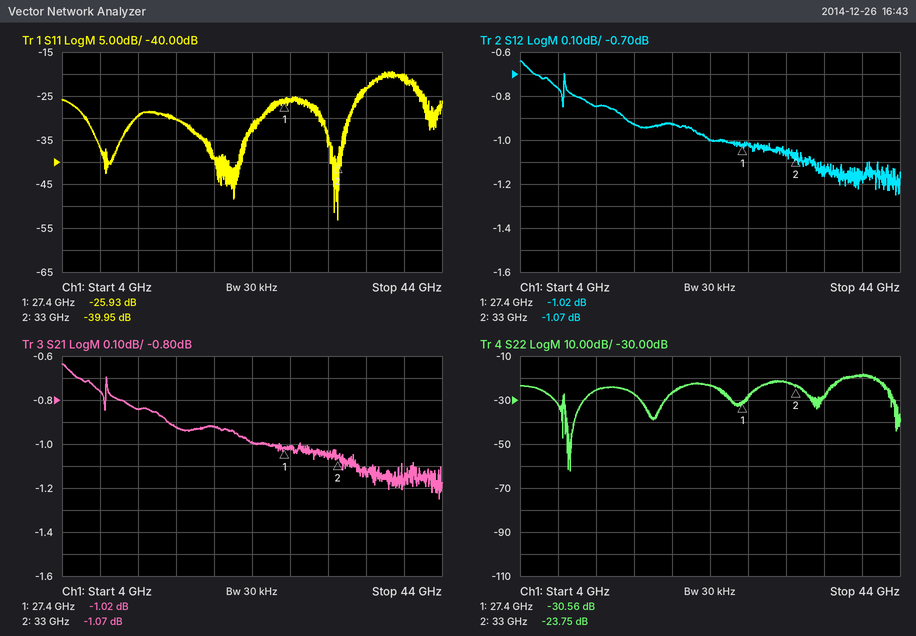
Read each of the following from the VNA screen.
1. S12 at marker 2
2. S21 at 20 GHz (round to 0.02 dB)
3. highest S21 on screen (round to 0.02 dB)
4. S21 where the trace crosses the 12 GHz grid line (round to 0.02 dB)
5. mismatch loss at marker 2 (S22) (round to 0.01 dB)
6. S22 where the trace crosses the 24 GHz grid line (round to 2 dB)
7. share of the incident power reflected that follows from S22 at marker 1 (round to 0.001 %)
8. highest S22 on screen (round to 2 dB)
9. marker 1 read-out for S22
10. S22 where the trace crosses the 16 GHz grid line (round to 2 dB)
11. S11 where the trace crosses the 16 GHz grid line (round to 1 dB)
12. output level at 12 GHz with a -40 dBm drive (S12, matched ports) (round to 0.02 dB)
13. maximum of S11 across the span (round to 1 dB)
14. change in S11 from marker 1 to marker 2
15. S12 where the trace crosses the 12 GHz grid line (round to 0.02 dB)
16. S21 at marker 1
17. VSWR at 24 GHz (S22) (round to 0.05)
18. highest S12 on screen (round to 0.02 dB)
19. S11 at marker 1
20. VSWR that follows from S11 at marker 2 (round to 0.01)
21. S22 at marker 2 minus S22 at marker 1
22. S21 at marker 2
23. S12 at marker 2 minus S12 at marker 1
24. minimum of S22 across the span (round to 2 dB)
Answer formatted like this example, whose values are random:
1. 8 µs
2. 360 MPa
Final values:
1. -1.07 dB
2. -0.92 dB
3. -0.64 dB
4. -0.84 dB
5. 0.02 dB
6. -24 dB
7. 0.088 %
8. -18 dB
9. -30.56 dB
10. -28 dB
11. -30 dB
12. -40.84 dBm
13. -19 dB
14. -14.02 dB
15. -0.84 dB
16. -1.02 dB
17. 1.15
18. -0.64 dB
19. -25.93 dB
20. 1.02
21. 6.81 dB
22. -1.07 dB
23. -0.05 dB
24. -62 dB
